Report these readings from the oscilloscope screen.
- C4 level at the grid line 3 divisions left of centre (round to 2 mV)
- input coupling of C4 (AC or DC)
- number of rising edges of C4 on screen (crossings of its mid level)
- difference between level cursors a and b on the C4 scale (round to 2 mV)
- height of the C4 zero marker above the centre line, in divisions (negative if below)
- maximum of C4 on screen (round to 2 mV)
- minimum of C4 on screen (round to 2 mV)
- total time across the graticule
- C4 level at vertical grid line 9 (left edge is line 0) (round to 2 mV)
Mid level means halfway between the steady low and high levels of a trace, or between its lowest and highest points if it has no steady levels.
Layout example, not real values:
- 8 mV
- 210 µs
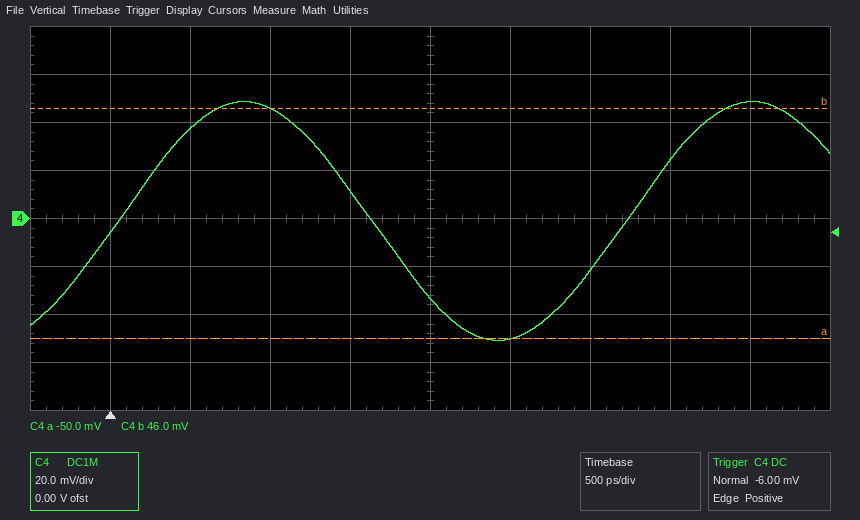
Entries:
- 38 mV
- DC
- 2
- 96 mV
- 0.0 div
- 48 mV
- -50 mV
- 5 ns
- 48 mV
